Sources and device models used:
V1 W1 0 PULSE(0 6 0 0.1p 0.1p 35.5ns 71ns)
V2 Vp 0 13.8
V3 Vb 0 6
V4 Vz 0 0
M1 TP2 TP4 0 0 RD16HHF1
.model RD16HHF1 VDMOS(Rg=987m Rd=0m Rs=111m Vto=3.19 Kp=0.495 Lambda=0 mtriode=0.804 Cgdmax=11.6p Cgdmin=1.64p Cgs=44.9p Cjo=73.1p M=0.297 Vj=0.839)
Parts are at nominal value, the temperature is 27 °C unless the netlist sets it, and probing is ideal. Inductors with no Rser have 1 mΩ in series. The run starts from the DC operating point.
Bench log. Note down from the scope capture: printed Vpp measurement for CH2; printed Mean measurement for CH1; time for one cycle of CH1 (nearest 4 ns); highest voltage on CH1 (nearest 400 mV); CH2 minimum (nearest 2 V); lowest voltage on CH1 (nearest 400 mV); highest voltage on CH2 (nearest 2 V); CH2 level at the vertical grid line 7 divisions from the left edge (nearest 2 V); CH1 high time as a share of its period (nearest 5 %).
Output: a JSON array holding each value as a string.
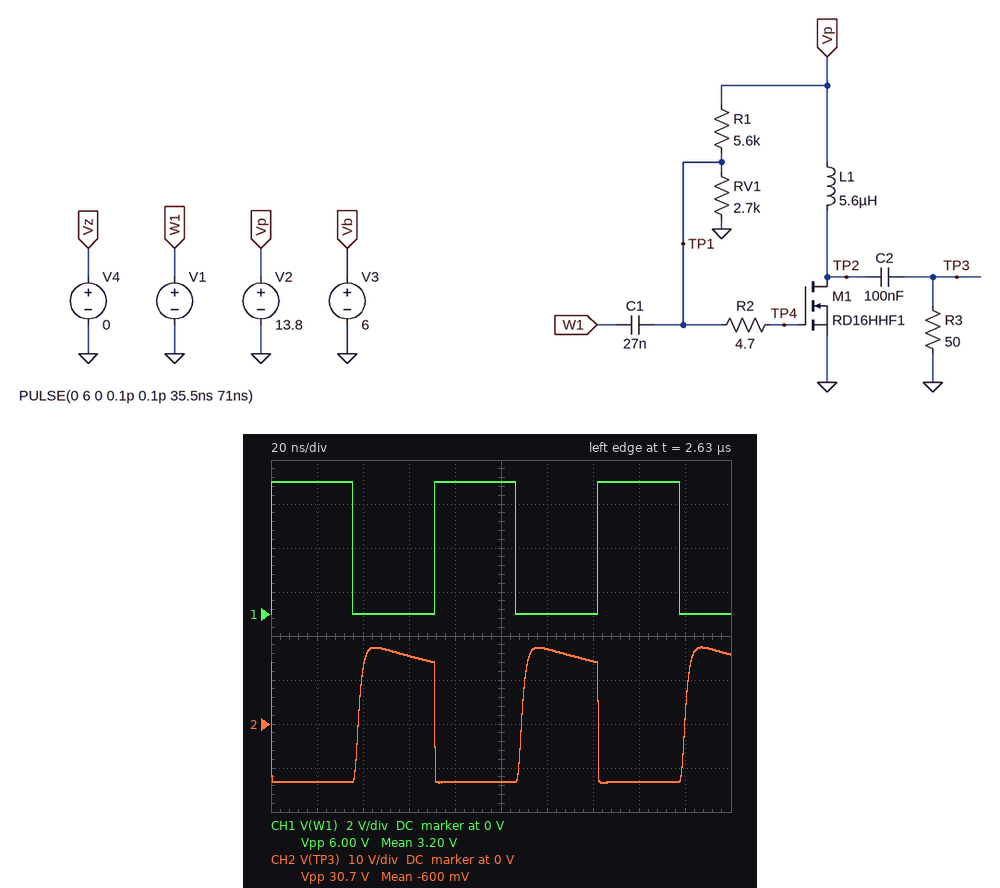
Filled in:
["30.7 V", "3.20 V", "72 ns", "6.0 V", "-14 V", "0 V", "18 V", "14 V", "50 %"]
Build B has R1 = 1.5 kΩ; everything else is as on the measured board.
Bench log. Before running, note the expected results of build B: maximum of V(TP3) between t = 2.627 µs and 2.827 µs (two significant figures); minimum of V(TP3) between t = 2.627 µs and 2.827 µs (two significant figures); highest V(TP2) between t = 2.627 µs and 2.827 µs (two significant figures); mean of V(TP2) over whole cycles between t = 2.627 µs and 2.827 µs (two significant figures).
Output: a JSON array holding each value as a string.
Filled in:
["18 V", "-12 V", "32 V", "15 V"]
